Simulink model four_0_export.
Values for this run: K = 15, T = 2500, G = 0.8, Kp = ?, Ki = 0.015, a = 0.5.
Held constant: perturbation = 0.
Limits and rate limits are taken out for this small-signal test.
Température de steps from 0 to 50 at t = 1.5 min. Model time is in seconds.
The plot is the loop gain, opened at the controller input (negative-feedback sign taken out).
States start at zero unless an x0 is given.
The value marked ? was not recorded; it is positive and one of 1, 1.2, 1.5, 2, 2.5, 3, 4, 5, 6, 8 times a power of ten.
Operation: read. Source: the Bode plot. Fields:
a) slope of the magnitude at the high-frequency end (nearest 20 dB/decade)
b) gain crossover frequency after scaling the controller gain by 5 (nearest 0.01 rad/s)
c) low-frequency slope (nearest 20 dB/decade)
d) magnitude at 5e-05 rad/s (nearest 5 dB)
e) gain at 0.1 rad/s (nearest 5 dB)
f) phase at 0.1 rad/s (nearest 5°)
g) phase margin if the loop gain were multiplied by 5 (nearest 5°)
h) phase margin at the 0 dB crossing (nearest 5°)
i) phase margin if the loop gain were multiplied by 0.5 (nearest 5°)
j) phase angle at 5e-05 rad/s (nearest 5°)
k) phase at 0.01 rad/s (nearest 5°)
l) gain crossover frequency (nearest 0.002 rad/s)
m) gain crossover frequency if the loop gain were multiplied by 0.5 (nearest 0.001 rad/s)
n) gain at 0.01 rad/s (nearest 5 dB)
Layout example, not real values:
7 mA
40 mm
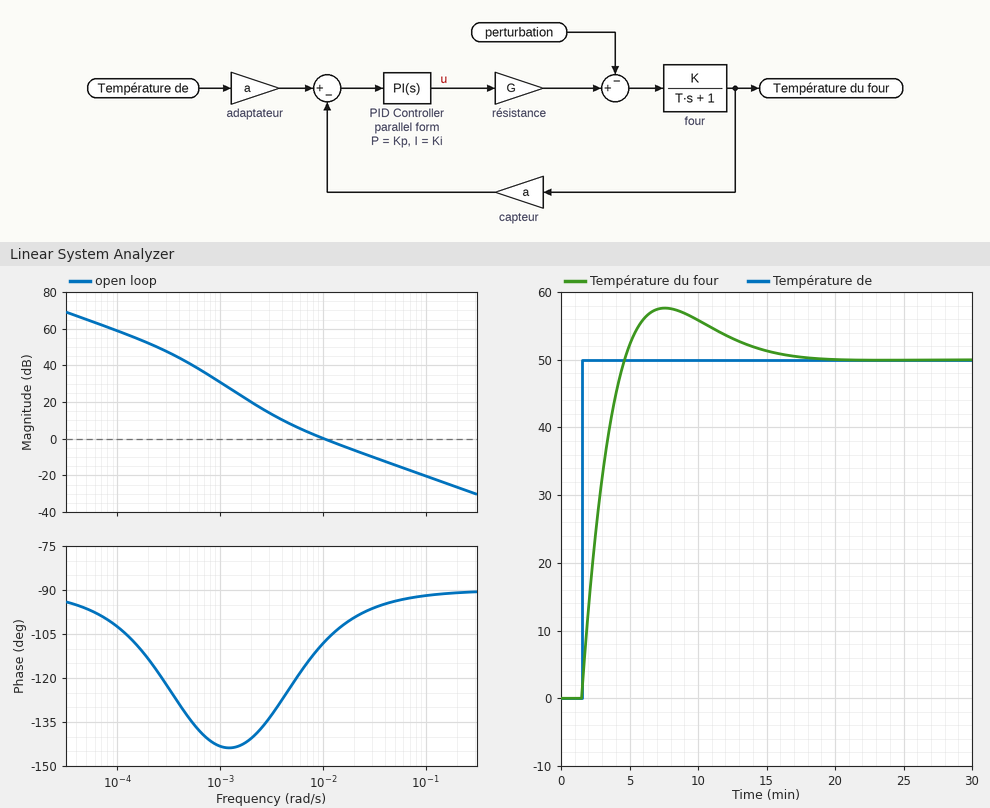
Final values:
-20 dB/decade
0.05 rad/s
-20 dB/decade
65 dB
-20 dB
-90°
85°
70°
60°
-95°
-110°
0.010 rad/s
0.006 rad/s
0 dB
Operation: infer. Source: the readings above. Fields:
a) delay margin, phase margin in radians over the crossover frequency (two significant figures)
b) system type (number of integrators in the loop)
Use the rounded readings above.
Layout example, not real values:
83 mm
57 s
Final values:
120 s
1
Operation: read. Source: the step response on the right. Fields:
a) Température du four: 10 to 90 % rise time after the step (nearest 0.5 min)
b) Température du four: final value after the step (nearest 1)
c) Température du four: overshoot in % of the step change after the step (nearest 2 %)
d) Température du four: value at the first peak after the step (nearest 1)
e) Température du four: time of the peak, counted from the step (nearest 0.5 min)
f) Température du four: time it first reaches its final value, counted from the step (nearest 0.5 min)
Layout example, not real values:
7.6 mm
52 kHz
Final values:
2.5 min
50
16 %
58
6.0 min
3.0 min
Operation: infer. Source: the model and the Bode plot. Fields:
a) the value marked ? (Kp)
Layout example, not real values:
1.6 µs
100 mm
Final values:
4
